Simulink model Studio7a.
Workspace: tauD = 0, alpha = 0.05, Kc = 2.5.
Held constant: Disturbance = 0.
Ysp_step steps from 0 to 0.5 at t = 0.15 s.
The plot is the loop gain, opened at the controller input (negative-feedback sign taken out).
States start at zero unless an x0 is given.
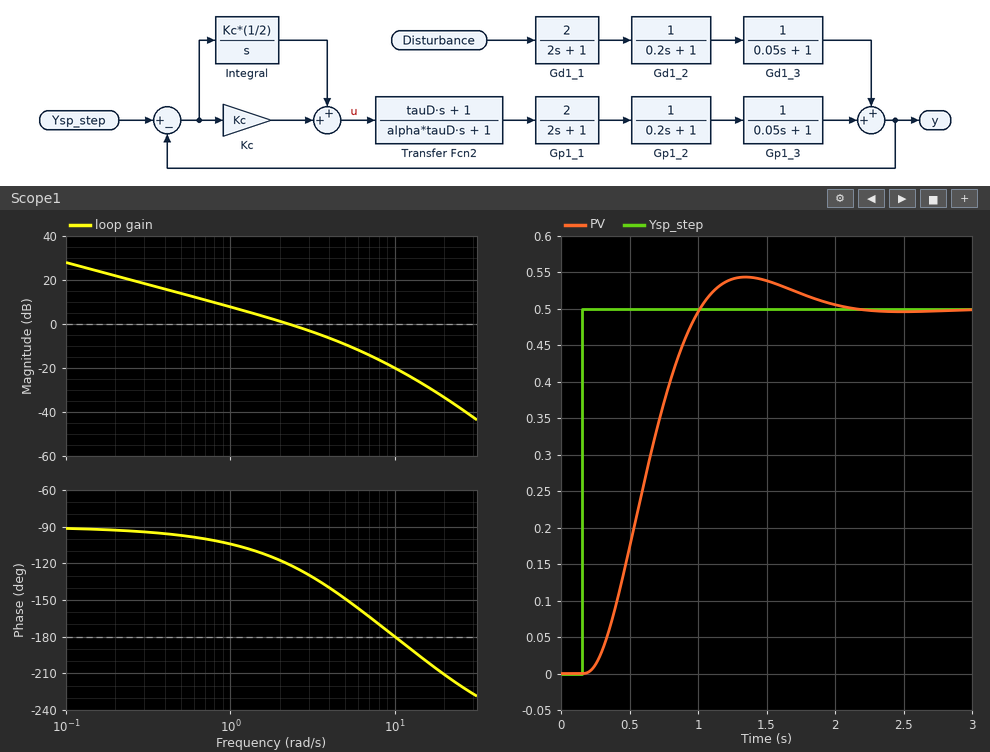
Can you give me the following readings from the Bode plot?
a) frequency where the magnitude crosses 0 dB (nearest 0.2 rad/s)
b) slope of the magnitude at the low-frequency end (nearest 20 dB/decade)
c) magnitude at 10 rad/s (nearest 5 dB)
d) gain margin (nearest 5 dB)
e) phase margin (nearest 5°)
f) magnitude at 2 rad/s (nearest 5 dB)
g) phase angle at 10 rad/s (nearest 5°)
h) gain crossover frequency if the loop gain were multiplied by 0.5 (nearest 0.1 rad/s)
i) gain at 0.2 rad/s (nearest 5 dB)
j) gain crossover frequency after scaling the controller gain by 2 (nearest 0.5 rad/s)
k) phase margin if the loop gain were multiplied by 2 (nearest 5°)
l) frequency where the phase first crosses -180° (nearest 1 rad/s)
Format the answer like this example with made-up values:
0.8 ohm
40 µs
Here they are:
2.2 rad/s
-20 dB/decade
-20 dB
20 dB
60°
0 dB
-180°
1.2 rad/s
20 dB
4.0 rad/s
40°
10 rad/s
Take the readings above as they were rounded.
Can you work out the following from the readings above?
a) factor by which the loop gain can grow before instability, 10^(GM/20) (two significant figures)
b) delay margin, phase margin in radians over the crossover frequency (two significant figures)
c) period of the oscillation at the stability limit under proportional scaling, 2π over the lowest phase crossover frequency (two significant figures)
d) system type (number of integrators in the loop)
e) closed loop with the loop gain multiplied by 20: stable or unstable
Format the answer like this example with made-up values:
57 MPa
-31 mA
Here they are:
10
0.48 s
0.63 s
1
unstable
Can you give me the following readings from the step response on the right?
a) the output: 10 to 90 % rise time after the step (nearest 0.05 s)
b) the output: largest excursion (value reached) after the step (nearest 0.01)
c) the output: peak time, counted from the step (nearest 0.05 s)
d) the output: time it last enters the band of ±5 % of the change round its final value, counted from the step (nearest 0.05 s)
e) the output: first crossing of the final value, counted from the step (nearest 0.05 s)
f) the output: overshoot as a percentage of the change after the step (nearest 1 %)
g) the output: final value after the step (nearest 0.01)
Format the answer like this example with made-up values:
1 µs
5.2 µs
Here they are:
0.55 s
0.54
1.20 s
1.55 s
0.85 s
9 %
0.50
